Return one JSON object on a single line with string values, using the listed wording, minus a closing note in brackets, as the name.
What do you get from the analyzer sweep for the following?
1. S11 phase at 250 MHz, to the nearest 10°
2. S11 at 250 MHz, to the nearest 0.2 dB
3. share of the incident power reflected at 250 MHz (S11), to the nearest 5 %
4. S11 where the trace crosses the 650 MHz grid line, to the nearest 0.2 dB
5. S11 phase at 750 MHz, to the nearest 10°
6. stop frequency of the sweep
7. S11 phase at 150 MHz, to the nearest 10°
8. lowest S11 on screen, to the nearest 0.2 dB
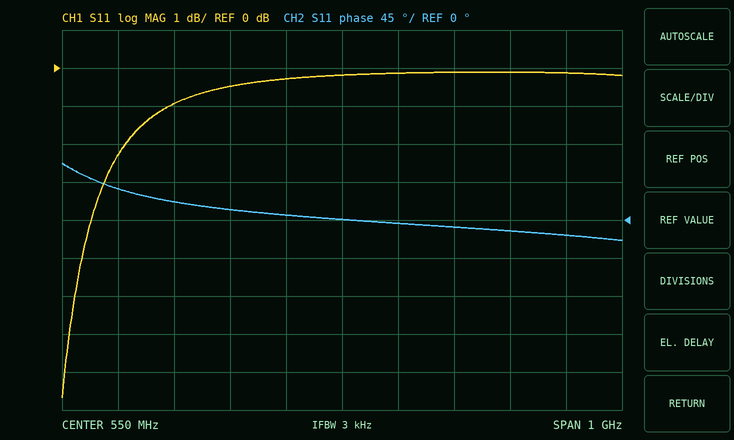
{"S11 phase at 250 MHz, to the nearest 10°": "20°", "S11 at 250 MHz, to the nearest 0.2 dB": "-1.0 dB", "share of the incident power reflected at 250 MHz (S11), to the nearest 5 %": "80 %", "S11 where the trace crosses the 650 MHz grid line, to the nearest 0.2 dB": "-0.2 dB", "S11 phase at 750 MHz, to the nearest 10°": "-10°", "stop frequency of the sweep": "1.05 GHz", "S11 phase at 150 MHz, to the nearest 10°": "40°", "lowest S11 on screen, to the nearest 0.2 dB": "-8.6 dB"}
